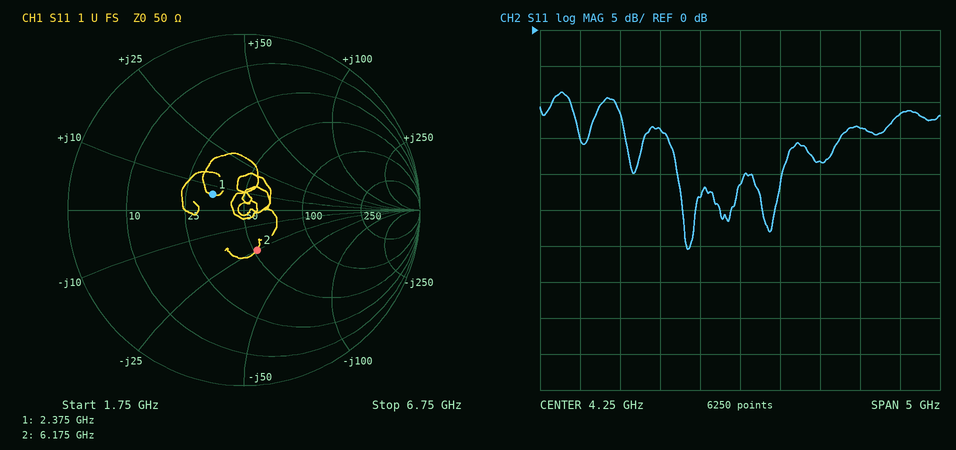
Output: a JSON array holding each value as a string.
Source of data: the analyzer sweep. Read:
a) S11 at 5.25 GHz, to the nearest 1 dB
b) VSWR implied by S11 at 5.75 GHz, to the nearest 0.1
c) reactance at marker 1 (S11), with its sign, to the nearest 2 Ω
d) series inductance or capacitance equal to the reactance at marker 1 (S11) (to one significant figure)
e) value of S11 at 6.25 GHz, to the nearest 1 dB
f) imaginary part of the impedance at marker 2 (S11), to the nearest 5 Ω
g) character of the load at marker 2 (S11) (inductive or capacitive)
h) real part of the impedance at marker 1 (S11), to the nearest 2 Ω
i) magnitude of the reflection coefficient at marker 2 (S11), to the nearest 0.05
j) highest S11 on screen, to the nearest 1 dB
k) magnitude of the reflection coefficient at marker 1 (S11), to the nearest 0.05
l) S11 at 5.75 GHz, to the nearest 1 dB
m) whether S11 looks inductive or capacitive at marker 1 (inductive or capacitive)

["-18 dB", "1.5", "+6 Ω", "400 pH", "-12 dB", "-25 Ω", "capacitive", "34 Ω", "0.25", "-9 dB", "0.20", "-14 dB", "inductive"]
